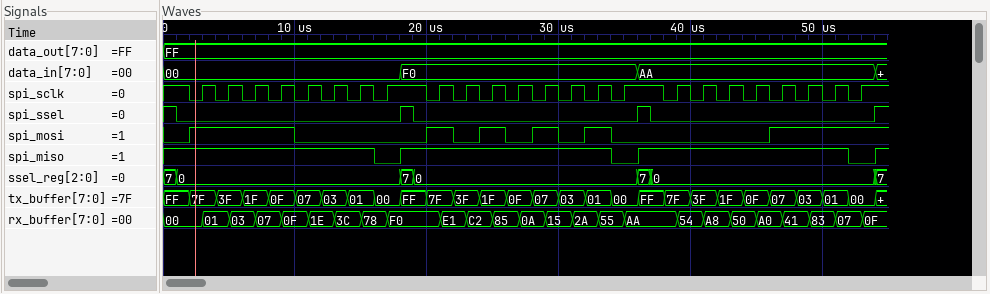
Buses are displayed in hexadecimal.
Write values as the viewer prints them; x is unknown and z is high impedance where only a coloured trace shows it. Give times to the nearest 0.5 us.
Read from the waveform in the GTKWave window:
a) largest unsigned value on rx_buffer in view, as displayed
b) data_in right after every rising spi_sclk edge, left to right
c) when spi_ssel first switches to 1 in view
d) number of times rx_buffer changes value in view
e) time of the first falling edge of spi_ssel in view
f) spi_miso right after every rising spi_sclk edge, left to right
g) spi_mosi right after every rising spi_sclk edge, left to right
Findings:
F0
00, 00, 00, 00, 00, 00, 00, 00, F0, F0, F0, F0, F0, F0, F0, F0, AA, AA, AA, AA, AA, AA, AA, AA
18 us
24
1 us
1 1 1 1 1 1 1 0 1 1 1 1 1 1 1 0 1 1 1 1 1 1 1 0
1 1 1 1 0 0 0 0 1 0 1 0 1 0 1 0 0 0 0 0 1 1 1 1
